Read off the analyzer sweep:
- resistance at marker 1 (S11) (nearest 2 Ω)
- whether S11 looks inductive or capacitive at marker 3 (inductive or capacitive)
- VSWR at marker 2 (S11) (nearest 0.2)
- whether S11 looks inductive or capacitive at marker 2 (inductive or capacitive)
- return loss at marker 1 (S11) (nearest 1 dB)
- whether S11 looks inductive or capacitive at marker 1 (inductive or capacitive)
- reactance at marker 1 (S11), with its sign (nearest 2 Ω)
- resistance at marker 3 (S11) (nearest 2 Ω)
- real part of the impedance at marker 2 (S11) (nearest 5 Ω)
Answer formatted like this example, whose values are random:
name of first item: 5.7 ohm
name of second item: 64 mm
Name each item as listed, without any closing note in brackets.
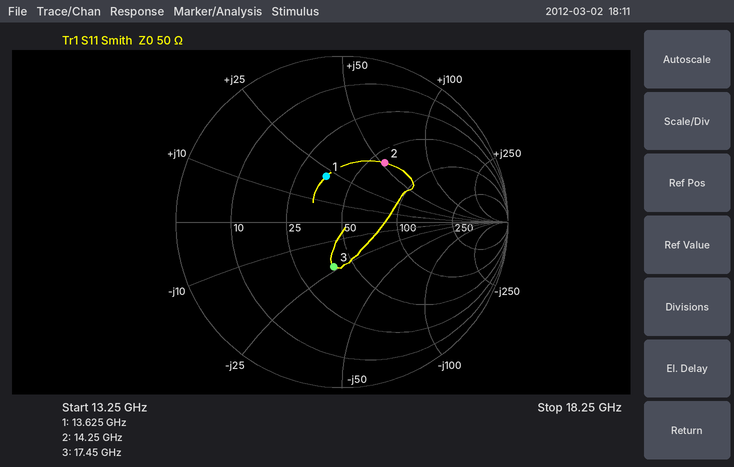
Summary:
resistance at marker 1 (S11): 36 Ω
whether S11 looks inductive or capacitive at marker 3: capacitive
VSWR at marker 2 (S11): 2.6
whether S11 looks inductive or capacitive at marker 2: inductive
return loss at marker 1 (S11): 11 dB
whether S11 looks inductive or capacitive at marker 1: inductive
reactance at marker 1 (S11), with its sign: +22 Ω
resistance at marker 3 (S11): 40 Ω
real part of the impedance at marker 2 (S11): 60 Ω
